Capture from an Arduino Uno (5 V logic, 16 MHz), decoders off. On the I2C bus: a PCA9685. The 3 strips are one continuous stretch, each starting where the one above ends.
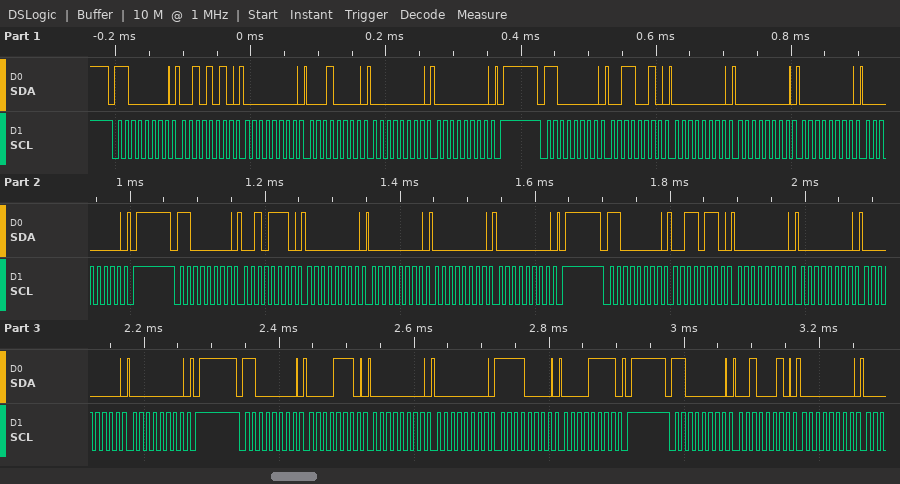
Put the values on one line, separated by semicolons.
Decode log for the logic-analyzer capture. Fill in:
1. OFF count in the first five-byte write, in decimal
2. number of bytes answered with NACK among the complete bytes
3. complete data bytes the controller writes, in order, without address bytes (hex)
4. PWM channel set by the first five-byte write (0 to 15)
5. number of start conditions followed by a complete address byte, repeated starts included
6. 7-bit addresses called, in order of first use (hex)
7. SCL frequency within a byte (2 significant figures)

0; 0; 2A 00 10 00 00 32 00 00 00 00 2E 00 00 00 00 36 00 00 00 00 0E 00 00 F0 0F 22 00; 9; 6; 0x60; 100 kHz
